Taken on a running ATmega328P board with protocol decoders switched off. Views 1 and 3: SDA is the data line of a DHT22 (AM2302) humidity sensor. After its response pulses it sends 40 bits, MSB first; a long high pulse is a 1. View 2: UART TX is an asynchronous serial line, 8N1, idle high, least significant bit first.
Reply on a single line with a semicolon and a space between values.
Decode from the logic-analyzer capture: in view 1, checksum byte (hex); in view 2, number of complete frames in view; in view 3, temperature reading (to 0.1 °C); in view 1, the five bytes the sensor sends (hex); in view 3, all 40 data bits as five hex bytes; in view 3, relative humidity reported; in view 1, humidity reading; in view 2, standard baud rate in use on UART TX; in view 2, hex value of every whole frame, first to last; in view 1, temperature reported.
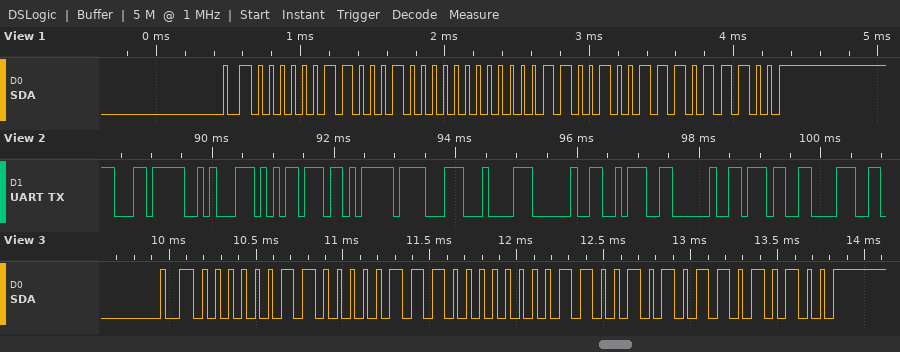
0xDC; 11; 20.2 °C; 03 10 00 C9 DC; 03 07 00 CA D4; 77.5 %; 78.4 %; 9600 baud; EC 8A B5 EB 8F 84 20 3A 20 37 38; 20.1 °C
